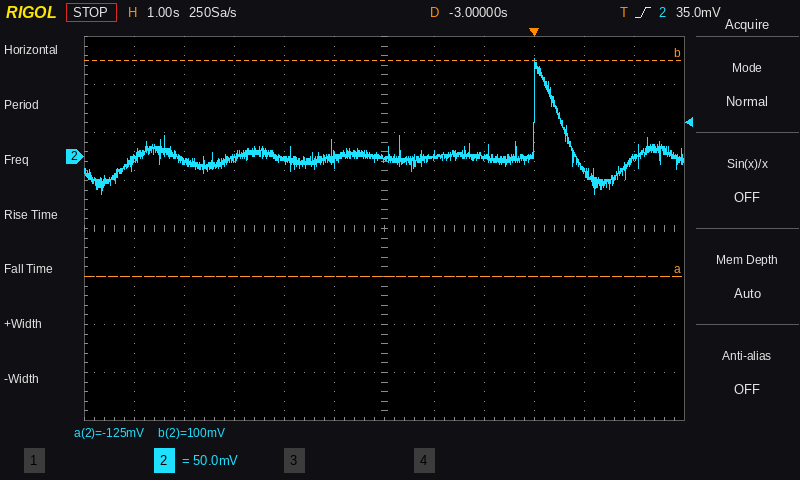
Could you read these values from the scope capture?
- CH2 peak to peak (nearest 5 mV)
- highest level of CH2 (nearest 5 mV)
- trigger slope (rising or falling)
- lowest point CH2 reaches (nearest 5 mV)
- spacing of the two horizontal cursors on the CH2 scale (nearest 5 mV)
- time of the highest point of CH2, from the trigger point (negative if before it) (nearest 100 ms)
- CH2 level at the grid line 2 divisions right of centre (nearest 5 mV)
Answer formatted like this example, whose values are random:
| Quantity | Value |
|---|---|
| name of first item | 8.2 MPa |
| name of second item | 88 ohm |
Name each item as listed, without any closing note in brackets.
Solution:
| Quantity | Value |
|---|---|
| CH2 peak to peak | 140 mV |
| highest level of CH2 | 100 mV |
| trigger slope | rising |
| lowest point CH2 reaches | -40 mV |
| spacing of the two horizontal cursors on the CH2 scale | 225 mV |
| time of the highest point of CH2, from the trigger point (negative if before it) | 0.0 s |
| CH2 level at the grid line 2 divisions right of centre | 0 mV |
